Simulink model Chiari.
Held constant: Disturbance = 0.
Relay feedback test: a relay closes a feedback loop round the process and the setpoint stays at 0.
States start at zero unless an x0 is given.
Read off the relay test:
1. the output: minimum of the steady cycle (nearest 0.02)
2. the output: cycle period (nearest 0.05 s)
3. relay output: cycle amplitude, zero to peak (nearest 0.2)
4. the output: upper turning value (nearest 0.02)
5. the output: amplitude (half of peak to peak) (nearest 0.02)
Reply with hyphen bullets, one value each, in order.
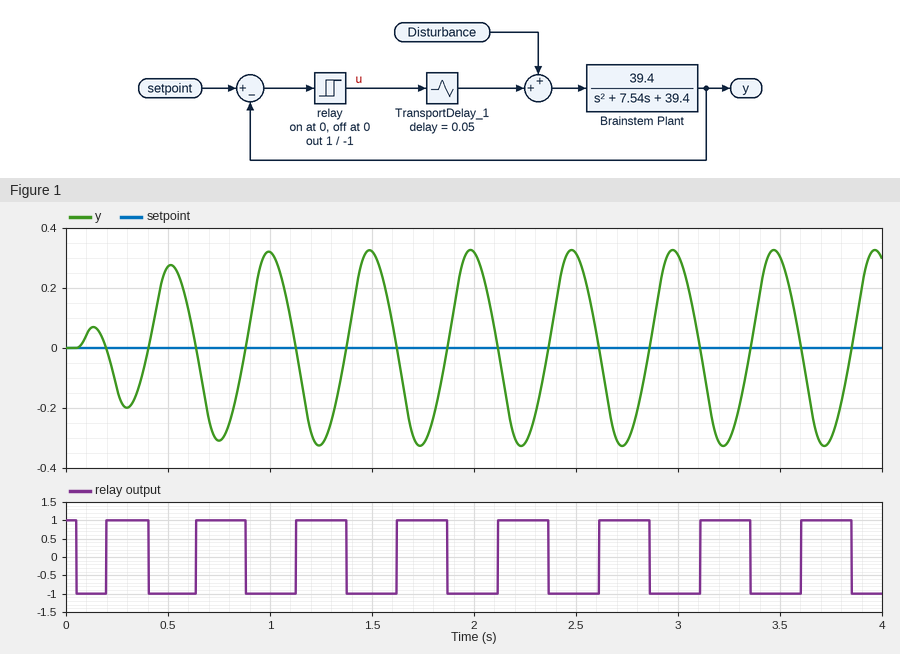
- -0.32
- 0.50 s
- 1.0
- 0.32
- 0.32
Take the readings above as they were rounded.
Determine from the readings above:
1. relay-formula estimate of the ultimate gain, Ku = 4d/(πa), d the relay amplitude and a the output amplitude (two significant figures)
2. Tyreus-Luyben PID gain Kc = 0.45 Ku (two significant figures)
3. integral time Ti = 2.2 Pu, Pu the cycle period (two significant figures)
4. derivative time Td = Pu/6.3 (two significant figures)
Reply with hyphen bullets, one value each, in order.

- 4.0
- 1.8
- 1.1 s
- 0.079 s
